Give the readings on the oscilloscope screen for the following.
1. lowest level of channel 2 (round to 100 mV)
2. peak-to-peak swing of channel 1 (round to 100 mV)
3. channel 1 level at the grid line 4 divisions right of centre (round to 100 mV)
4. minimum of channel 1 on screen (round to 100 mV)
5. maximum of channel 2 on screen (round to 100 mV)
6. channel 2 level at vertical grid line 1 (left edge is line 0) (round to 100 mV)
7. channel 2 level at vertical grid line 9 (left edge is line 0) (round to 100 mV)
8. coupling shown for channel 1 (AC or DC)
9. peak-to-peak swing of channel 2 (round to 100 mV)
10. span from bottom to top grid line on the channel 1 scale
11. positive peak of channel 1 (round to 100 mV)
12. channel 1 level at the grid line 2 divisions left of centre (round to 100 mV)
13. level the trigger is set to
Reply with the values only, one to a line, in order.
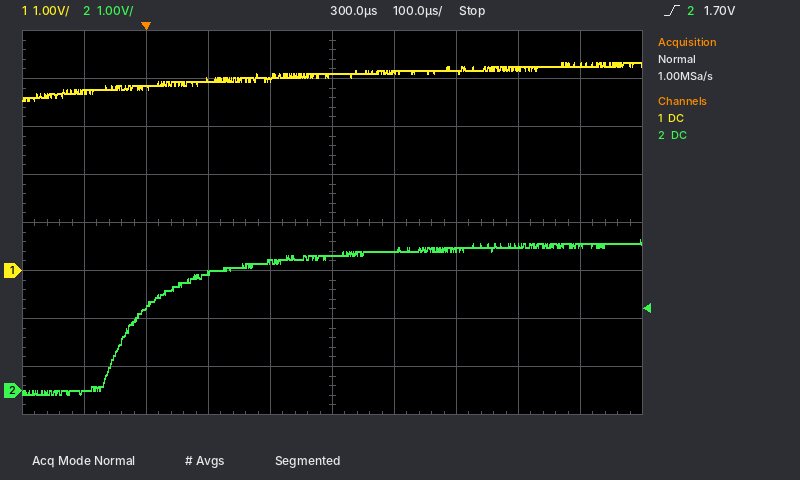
-100 mV
800 mV
4.3 V
3.5 V
3.1 V
0.0 V
3.0 V
DC
3.2 V
8 V
4.3 V
4.0 V
1.70 V
